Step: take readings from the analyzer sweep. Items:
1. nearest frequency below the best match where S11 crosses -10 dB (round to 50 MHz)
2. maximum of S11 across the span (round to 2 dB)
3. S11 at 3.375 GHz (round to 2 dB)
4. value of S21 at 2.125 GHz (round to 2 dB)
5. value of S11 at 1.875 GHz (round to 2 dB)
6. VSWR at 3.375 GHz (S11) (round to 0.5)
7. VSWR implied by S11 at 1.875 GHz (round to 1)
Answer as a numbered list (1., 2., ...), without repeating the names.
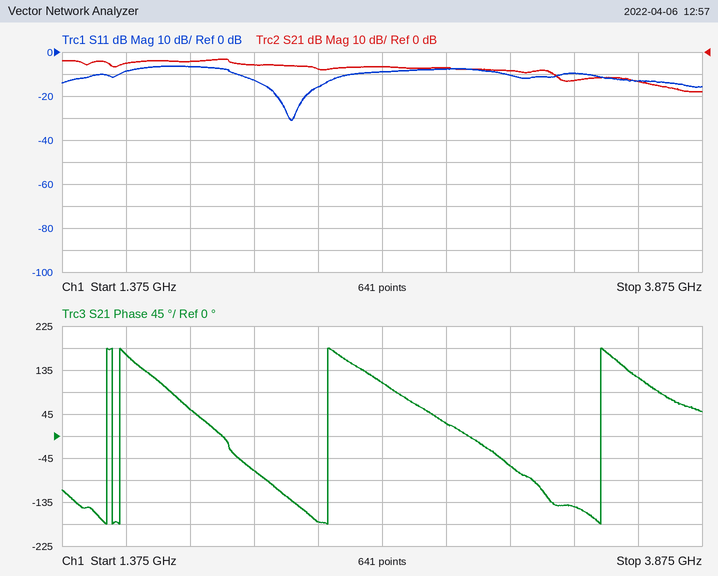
1. 2.05 GHz
2. -6 dB
3. -10 dB
4. -6 dB
5. -6 dB
6. 2.0
7. 3
